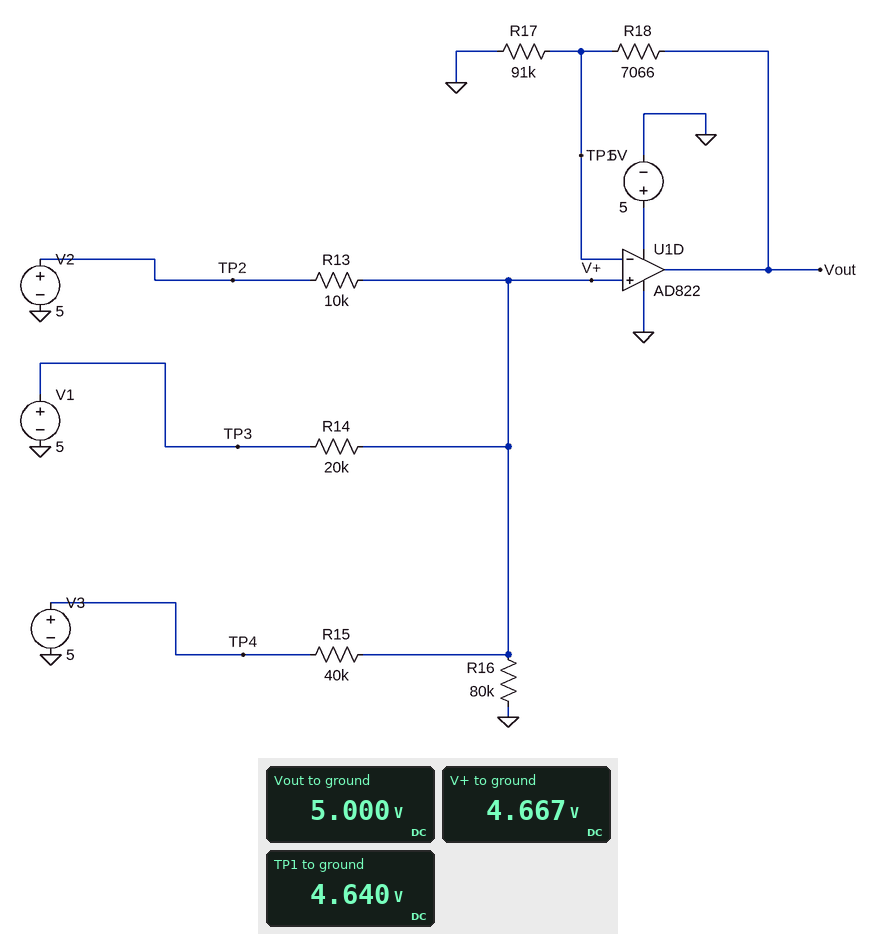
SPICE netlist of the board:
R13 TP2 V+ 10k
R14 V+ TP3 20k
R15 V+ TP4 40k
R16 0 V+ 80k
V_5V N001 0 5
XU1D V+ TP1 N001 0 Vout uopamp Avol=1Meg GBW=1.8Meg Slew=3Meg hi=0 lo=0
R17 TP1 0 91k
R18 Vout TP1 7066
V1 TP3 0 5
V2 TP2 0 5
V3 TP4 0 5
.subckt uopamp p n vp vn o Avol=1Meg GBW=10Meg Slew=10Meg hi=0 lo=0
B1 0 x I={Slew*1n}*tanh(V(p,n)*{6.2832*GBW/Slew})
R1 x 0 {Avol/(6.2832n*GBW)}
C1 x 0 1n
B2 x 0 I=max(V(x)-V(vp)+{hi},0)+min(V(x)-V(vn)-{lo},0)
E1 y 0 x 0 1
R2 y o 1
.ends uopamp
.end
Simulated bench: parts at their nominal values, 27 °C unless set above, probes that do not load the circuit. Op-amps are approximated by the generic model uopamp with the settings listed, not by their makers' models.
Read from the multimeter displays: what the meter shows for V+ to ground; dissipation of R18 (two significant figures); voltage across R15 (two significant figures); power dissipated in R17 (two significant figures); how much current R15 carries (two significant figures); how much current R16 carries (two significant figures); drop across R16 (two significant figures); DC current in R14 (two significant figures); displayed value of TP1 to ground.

4.667 V
18 µW
330 mV
240 µW
8.3 µA
58 µA
4.7 V
17 µA
4.640 V
